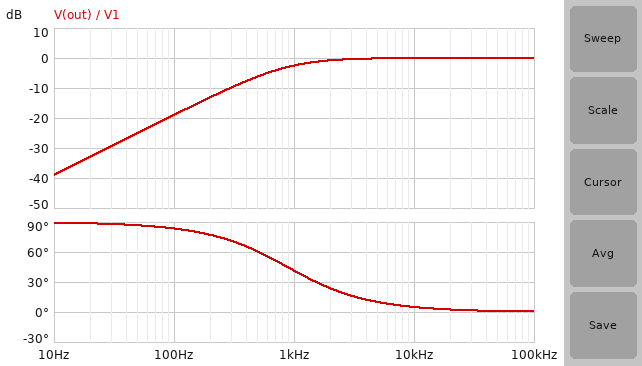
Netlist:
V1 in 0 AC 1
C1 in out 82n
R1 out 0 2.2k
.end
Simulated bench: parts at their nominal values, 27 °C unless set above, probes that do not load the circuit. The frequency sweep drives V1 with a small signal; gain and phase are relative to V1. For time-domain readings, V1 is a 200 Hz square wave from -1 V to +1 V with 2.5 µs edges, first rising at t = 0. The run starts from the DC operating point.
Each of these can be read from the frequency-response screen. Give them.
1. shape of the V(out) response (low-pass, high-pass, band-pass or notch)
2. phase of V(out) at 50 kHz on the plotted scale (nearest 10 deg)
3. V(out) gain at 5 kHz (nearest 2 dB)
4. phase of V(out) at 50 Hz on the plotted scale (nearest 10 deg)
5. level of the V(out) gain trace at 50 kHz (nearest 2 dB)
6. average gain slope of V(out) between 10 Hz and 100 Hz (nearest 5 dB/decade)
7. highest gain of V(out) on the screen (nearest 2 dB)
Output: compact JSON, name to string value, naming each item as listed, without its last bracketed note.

{"shape of the V(out) response": "high-pass", "phase of V(out) at 50 kHz on the plotted scale": "0 deg", "V(out) gain at 5 kHz": "0 dB", "phase of V(out) at 50 Hz on the plotted scale": "90 deg", "level of the V(out) gain trace at 50 kHz": "0 dB", "average gain slope of V(out) between 10 Hz and 100 Hz": "20 dB/decade", "highest gain of V(out) on the screen": "0 dB"}
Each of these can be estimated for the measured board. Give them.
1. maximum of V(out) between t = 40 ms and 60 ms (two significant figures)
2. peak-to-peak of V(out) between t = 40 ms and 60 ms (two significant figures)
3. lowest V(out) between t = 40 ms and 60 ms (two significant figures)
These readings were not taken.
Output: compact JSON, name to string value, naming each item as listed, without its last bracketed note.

{"maximum of V(out) between t = 40 ms and 60 ms": "2.0 V", "peak-to-peak of V(out) between t = 40 ms and 60 ms": "4.0 V", "lowest V(out) between t = 40 ms and 60 ms": "-2.0 V"}
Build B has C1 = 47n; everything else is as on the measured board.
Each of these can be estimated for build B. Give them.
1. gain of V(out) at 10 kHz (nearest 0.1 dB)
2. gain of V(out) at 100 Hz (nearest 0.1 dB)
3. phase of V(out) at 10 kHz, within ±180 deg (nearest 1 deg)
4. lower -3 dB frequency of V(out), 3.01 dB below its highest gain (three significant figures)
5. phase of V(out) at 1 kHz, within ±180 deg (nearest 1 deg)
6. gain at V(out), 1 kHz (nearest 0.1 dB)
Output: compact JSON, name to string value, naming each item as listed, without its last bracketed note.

{"gain of V(out) at 10 kHz": "-0.1 dB", "gain of V(out) at 100 Hz": "-23.8 dB", "phase of V(out) at 10 kHz, within ±180 deg": "9 deg", "lower -3 dB frequency of V(out), 3.01 dB below its highest gain": "1.54 kHz", "phase of V(out) at 1 kHz, within ±180 deg": "57 deg", "gain at V(out), 1 kHz": "-5.3 dB"}
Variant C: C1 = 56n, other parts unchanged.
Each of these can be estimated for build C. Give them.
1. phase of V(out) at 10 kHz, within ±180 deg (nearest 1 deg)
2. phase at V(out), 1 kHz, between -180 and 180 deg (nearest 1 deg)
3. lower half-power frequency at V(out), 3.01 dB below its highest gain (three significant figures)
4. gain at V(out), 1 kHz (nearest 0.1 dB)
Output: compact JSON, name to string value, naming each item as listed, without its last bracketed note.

{"phase of V(out) at 10 kHz, within ±180 deg": "7 deg", "phase at V(out), 1 kHz, between -180 and 180 deg": "52 deg", "lower half-power frequency at V(out), 3.01 dB below its highest gain": "1.29 kHz", "gain at V(out), 1 kHz": "-4.3 dB"}
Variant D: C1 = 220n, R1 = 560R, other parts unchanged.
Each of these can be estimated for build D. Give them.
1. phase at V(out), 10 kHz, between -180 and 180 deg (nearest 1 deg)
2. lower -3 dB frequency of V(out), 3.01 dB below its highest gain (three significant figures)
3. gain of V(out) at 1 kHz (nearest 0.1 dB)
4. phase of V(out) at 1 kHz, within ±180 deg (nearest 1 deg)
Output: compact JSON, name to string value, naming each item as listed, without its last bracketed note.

{"phase at V(out), 10 kHz, between -180 and 180 deg": "7 deg", "lower -3 dB frequency of V(out), 3.01 dB below its highest gain": "1.29 kHz", "gain of V(out) at 1 kHz": "-4.3 dB", "phase of V(out) at 1 kHz, within ±180 deg": "52 deg"}
